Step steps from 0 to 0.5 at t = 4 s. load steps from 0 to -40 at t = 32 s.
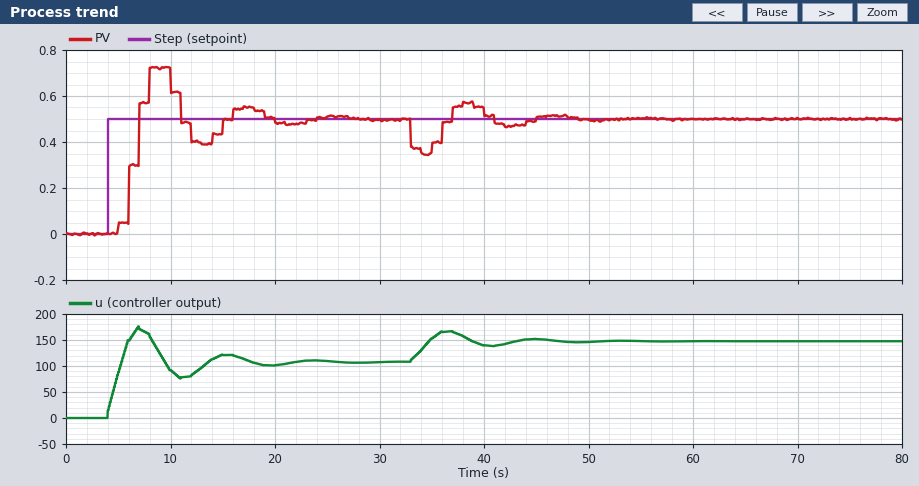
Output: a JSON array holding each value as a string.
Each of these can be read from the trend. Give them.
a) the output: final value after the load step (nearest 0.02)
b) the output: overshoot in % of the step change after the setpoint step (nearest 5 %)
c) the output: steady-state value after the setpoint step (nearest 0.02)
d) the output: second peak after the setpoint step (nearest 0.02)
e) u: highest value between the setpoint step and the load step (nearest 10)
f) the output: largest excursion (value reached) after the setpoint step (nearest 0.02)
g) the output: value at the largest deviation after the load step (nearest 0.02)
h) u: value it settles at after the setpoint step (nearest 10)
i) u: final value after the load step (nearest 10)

["0.50", "45 %", "0.50", "0.56", "180", "0.72", "0.34", "110", "150"]
